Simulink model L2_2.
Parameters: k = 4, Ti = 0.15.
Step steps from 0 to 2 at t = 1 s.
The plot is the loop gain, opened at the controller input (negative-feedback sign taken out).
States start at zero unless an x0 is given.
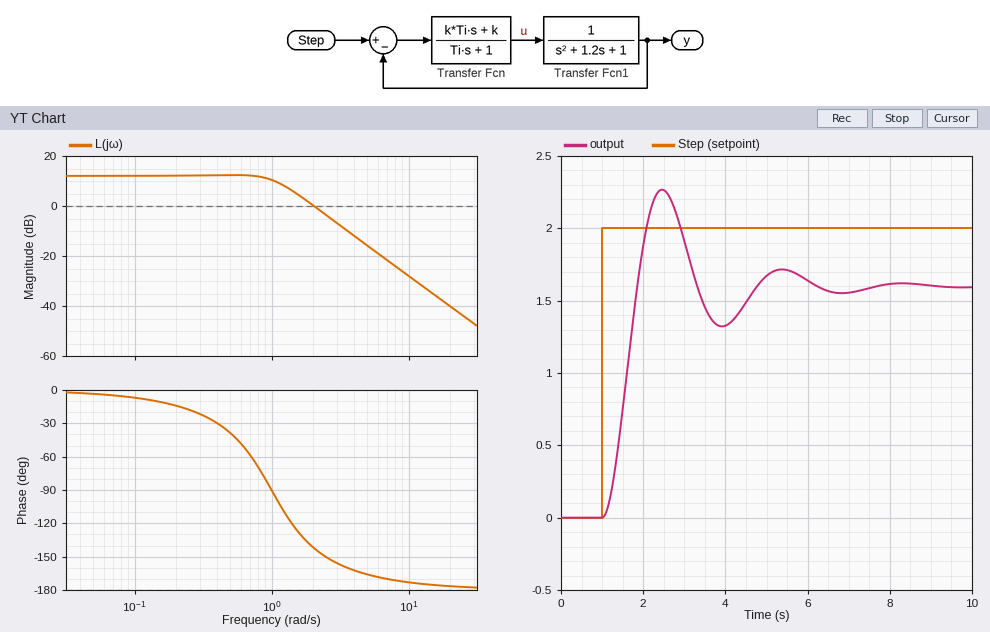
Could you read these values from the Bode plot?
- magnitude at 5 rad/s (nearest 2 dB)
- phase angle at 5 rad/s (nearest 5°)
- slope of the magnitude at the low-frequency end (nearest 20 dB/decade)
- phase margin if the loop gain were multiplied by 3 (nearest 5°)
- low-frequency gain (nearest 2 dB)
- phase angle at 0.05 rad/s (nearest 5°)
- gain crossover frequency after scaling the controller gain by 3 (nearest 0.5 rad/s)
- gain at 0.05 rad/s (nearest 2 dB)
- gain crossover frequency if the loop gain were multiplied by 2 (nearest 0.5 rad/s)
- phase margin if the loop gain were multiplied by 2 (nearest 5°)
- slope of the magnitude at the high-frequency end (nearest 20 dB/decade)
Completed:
-16 dB
-165°
0 dB/decade
20°
12 dB
-5°
3.5 rad/s
12 dB
3.0 rad/s
25°
-40 dB/decade
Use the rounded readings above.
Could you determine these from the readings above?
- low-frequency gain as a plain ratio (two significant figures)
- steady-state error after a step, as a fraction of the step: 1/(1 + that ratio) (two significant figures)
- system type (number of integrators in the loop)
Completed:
4.0
0.20
0
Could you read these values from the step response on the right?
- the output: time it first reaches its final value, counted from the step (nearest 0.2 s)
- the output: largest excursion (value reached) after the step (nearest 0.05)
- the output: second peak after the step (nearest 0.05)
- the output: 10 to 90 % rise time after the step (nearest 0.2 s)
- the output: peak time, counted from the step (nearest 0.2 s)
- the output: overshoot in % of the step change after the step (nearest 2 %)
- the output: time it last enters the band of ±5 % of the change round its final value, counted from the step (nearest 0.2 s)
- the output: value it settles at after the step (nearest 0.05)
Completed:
0.8 s
2.25
1.70
0.6 s
1.4 s
42 %
4.8 s
1.60
